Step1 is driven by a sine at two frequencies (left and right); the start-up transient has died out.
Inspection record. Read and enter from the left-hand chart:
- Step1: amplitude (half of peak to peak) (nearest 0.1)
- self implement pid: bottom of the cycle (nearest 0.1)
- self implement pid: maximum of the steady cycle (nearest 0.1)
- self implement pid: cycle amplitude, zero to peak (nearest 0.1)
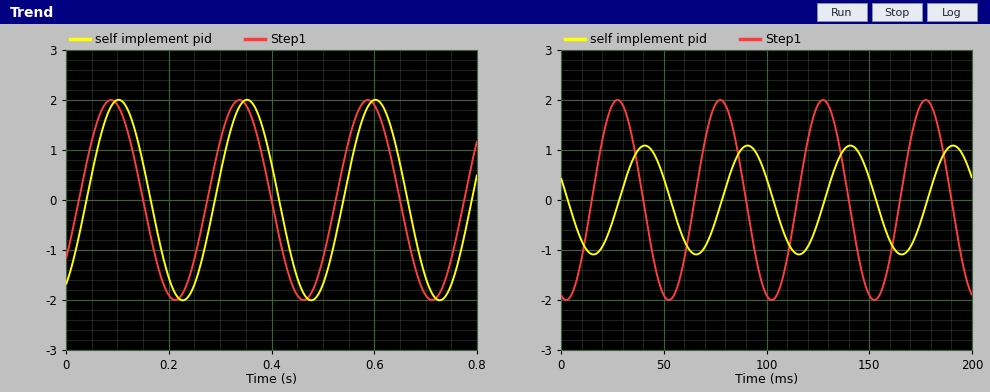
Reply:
2.0
-2.0
2.0
2.0
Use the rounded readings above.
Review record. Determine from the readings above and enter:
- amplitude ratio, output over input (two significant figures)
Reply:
1.0
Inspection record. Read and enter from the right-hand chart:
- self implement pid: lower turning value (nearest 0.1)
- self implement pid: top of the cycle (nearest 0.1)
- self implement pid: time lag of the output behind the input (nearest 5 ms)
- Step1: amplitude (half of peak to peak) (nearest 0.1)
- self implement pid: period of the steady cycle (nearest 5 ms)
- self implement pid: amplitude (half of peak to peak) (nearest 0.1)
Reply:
-1.1
1.1
15 ms
2.0
50 ms
1.1
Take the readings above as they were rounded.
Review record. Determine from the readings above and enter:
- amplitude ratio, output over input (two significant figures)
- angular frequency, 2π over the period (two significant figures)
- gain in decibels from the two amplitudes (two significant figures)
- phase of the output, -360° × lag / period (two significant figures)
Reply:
0.55
0.13 rad/ms
-5.2 dB
-110°
